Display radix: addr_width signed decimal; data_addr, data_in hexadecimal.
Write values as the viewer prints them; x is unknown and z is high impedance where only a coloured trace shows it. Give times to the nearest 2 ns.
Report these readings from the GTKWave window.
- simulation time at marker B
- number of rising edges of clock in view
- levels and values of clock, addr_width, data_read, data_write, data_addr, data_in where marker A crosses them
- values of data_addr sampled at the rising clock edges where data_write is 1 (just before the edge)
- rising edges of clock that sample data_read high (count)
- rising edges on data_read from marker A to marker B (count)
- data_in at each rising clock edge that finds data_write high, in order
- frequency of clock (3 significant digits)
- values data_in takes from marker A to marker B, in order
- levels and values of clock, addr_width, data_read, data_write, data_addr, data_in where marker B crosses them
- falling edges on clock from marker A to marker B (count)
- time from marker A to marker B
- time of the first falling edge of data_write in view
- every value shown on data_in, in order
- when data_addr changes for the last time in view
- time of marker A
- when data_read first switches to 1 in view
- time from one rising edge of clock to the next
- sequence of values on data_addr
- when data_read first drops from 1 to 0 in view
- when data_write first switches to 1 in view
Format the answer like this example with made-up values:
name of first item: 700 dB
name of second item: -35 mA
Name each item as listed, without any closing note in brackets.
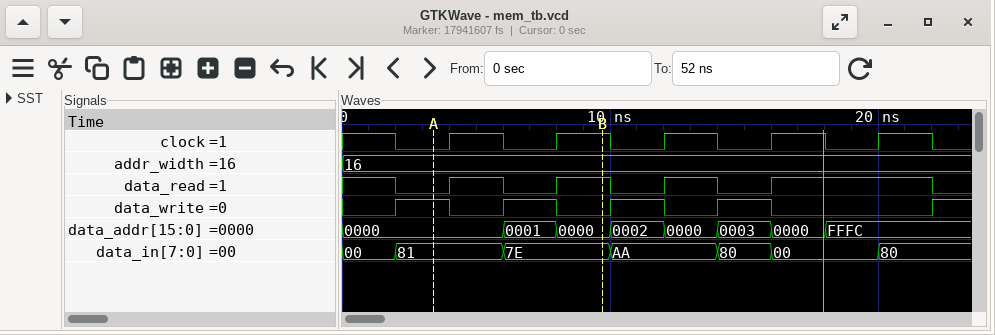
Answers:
simulation time at marker B: 10 ns
number of rising edges of clock in view: 5
levels and values of clock, addr_width, data_read, data_write, data_addr, data_in where marker A crosses them: clock=0, addr_width=16, data_read=0, data_write=1, data_addr=0000, data_in=81
values of data_addr sampled at the rising clock edges where data_write is 1: 0000, 0001, 0002, 0003
rising edges of clock that sample data_read high: 1
rising edges on data_read from marker A to marker B: 2
data_in at each rising clock edge that finds data_write high, in order: 81, 7E, AA, 80
frequency of clock: 250 MHz
values data_in takes from marker A to marker B, in order: 81, 7E
levels and values of clock, addr_width, data_read, data_write, data_addr, data_in where marker B crosses them: clock=1, addr_width=16, data_read=1, data_write=0, data_addr=0000, data_in=7E
falling edges on clock from marker A to marker B: 1
time from marker A to marker B: 6 ns
time of the first falling edge of data_write in view: 4 ns
every value shown on data_in, in order: 00, 81, 7E, AA, 80, 00, 80
when data_addr changes for the last time in view: 18 ns
time of marker A: 4 ns
when data_read first switches to 1 in view: 4 ns
time from one rising edge of clock to the next: 4 ns
sequence of values on data_addr: 0000, 0001, 0000, 0002, 0000, 0003, 0000, FFFC
when data_read first drops from 1 to 0 in view: 2 ns
when data_write first switches to 1 in view: 2 ns
